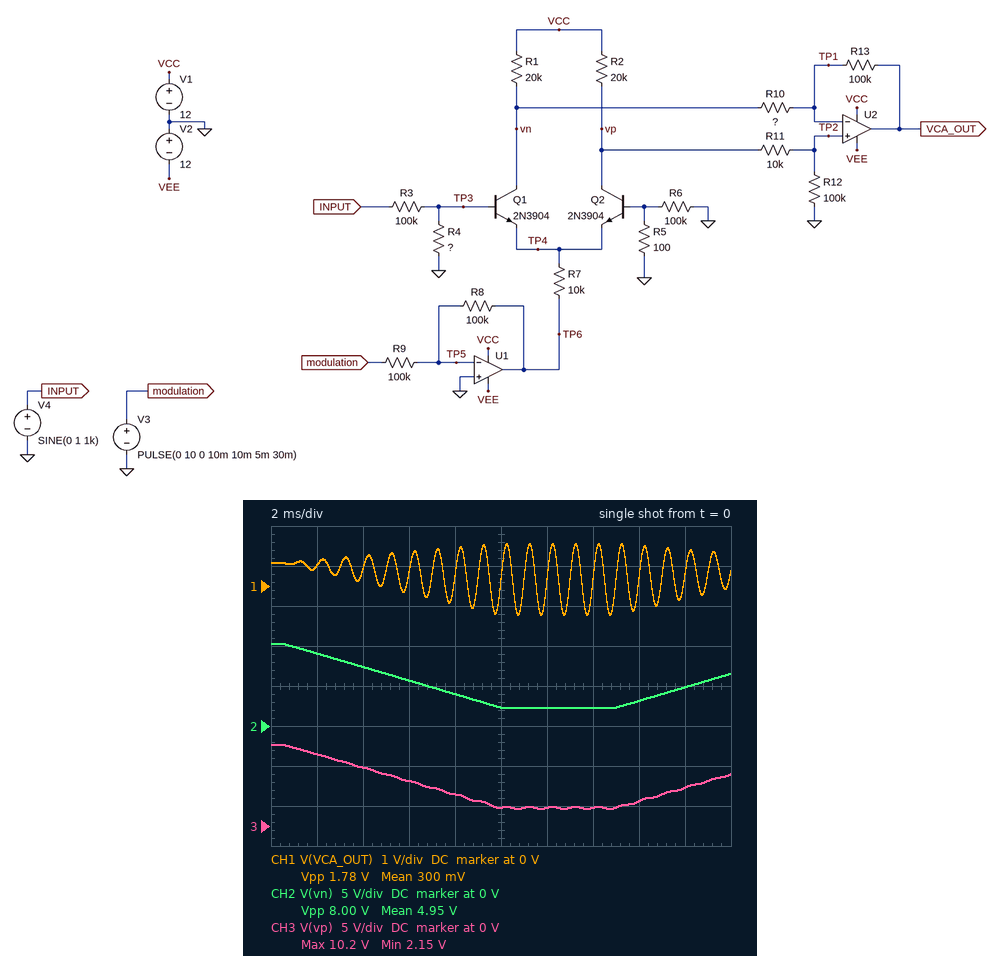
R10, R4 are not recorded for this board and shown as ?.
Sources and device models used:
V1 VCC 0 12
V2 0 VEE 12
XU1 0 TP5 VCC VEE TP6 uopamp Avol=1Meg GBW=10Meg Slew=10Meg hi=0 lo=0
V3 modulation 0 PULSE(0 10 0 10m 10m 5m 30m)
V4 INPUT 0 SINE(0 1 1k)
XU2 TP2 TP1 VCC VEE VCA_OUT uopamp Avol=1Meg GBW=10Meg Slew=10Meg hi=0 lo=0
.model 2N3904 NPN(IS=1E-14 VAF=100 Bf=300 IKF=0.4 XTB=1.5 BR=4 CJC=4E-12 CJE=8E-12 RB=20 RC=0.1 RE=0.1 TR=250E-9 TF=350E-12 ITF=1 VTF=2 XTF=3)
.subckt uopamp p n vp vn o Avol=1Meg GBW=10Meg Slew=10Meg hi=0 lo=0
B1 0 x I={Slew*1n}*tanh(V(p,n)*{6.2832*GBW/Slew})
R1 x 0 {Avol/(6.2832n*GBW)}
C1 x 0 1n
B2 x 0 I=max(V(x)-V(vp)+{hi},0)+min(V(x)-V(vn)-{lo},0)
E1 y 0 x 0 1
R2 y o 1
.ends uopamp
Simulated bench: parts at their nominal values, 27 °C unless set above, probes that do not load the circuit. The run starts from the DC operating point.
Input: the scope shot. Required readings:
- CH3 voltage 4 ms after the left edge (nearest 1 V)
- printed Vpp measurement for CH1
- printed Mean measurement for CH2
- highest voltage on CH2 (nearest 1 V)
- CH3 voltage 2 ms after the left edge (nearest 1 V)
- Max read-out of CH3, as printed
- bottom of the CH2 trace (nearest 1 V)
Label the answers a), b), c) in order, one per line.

a) 7 V
b) 1.78 V
c) 4.95 V
d) 10 V
e) 9 V
f) 10.2 V
g) 2 V
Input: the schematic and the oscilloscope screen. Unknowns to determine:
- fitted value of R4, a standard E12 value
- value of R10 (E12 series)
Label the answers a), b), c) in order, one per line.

a) 82 Ω
b) 12 kΩ
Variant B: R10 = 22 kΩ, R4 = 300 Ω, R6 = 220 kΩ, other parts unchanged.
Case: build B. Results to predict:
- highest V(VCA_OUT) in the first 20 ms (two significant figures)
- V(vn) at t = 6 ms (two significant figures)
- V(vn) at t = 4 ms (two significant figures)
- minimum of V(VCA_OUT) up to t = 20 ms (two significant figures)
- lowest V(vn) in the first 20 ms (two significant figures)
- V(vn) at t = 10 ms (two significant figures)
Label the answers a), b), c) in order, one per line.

a) 2.9 V
b) 5.9 V
c) 7.7 V
d) -2.2 V
e) 2.3 V
f) 2.4 V
